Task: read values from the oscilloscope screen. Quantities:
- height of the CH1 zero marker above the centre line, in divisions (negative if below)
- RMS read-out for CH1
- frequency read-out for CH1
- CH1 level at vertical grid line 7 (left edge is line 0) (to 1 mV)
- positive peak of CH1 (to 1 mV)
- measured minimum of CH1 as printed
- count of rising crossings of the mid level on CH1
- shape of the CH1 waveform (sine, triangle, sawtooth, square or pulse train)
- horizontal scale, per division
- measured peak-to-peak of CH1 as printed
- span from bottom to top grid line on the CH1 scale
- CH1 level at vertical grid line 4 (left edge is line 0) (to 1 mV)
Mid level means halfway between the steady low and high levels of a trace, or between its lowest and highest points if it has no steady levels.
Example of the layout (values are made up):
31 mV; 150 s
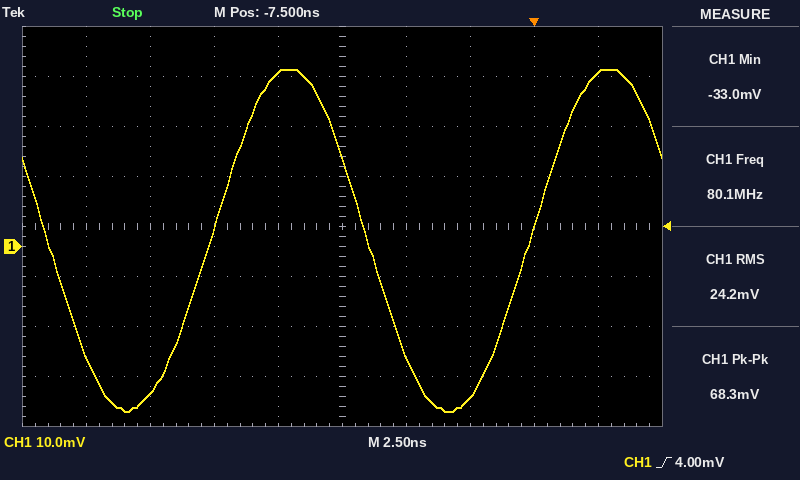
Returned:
-0.4 div; 24.2 mV; 80.1 MHz; -30 mV; 35 mV; -33.0 mV; 2; sine; 2.5 ns; 68.3 mV; 80 mV; 35 mV
